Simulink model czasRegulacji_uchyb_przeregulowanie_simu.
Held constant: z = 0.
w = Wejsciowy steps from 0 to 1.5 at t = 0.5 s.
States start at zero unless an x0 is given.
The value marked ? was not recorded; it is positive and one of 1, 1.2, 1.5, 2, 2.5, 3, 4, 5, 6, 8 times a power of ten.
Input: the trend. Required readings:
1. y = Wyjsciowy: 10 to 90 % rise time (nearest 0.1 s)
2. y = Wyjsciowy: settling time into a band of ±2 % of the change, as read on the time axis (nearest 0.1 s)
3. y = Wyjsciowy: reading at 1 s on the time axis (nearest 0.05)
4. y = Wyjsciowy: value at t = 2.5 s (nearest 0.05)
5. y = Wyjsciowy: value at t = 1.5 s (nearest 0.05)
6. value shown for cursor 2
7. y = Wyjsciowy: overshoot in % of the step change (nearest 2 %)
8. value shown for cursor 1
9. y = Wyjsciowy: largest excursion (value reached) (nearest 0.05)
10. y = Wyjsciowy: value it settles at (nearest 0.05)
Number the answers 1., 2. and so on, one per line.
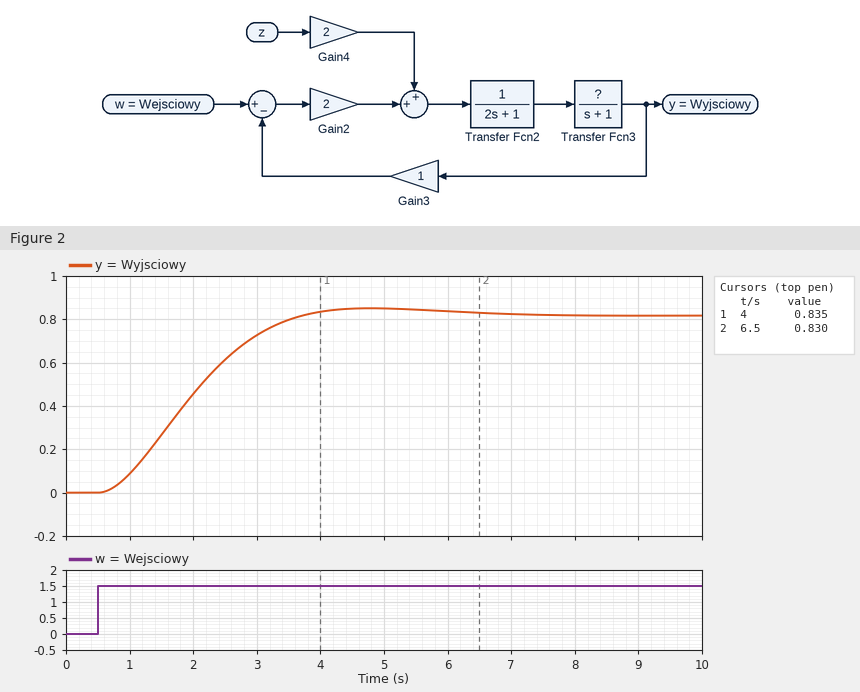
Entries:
1. 2.1 s
2. 6.2 s
3. 0.10
4. 0.60
5. 0.25
6. 0.830
7. 4 %
8. 0.835
9. 0.85
10. 0.80
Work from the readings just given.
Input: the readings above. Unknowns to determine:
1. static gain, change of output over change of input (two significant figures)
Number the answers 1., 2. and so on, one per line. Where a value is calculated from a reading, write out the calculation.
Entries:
1. (0.8 - 0) / (1.5 - 0) = 0.53
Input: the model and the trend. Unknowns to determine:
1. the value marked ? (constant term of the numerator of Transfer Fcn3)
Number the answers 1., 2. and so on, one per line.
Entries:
1. 0.6
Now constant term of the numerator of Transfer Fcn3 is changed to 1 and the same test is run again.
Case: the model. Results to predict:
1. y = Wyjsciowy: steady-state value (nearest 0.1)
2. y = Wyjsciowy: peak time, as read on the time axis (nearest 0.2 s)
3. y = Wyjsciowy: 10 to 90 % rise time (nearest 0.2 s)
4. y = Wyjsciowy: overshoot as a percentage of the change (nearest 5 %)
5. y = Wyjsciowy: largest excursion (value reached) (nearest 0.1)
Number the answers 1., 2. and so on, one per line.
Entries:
1. 1.0
2. 3.8 s
3. 1.6 s
4. 10 %
5. 1.1
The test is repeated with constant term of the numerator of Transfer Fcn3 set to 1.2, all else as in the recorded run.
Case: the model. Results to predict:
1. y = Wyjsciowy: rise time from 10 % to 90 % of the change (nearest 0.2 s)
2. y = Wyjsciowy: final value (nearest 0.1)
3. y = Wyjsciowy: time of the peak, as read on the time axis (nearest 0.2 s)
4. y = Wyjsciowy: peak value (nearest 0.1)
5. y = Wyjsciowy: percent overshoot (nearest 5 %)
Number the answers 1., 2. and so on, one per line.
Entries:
1. 1.4 s
2. 1.1
3. 3.4 s
4. 1.2
5. 10 %
